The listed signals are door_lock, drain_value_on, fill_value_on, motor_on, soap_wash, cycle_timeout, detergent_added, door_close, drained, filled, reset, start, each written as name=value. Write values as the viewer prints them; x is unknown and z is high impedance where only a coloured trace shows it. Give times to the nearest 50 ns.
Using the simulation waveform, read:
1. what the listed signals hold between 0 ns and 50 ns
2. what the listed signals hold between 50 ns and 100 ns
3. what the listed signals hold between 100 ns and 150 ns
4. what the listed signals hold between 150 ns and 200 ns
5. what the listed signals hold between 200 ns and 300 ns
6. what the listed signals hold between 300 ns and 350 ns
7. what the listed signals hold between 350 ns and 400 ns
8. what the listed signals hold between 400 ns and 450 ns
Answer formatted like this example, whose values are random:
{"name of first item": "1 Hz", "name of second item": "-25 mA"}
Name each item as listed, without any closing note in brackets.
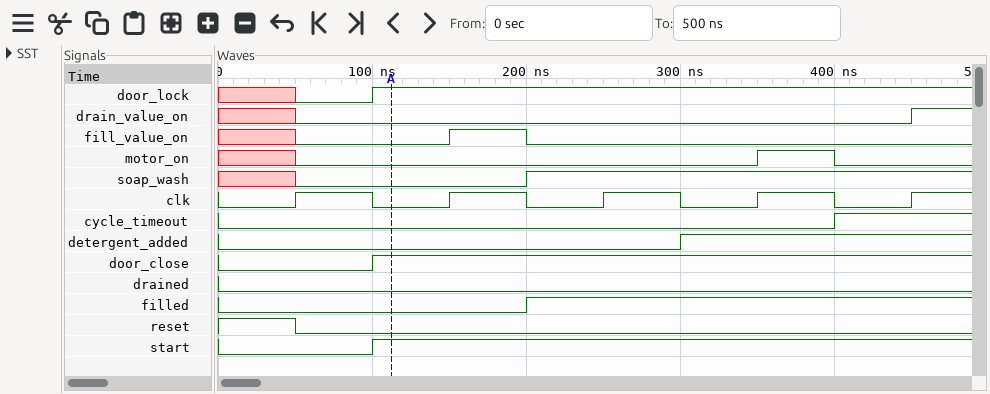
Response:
{"what the listed signals hold between 0 ns and 50 ns": "door_lock=x, drain_value_on=x, fill_value_on=x, motor_on=x, soap_wash=x, cycle_timeout=0, detergent_added=0, door_close=0, drained=0, filled=0, reset=1, start=0", "what the listed signals hold between 50 ns and 100 ns": "door_lock=0, drain_value_on=0, fill_value_on=0, motor_on=0, soap_wash=0, cycle_timeout=0, detergent_added=0, door_close=0, drained=0, filled=0, reset=0, start=0", "what the listed signals hold between 100 ns and 150 ns": "door_lock=1, drain_value_on=0, fill_value_on=0, motor_on=0, soap_wash=0, cycle_timeout=0, detergent_added=0, door_close=1, drained=0, filled=0, reset=0, start=1", "what the listed signals hold between 150 ns and 200 ns": "door_lock=1, drain_value_on=0, fill_value_on=1, motor_on=0, soap_wash=0, cycle_timeout=0, detergent_added=0, door_close=1, drained=0, filled=0, reset=0, start=1", "what the listed signals hold between 200 ns and 300 ns": "door_lock=1, drain_value_on=0, fill_value_on=0, motor_on=0, soap_wash=1, cycle_timeout=0, detergent_added=0, door_close=1, drained=0, filled=1, reset=0, start=1", "what the listed signals hold between 300 ns and 350 ns": "door_lock=1, drain_value_on=0, fill_value_on=0, motor_on=0, soap_wash=1, cycle_timeout=0, detergent_added=1, door_close=1, drained=0, filled=1, reset=0, start=1", "what the listed signals hold between 350 ns and 400 ns": "door_lock=1, drain_value_on=0, fill_value_on=0, motor_on=1, soap_wash=1, cycle_timeout=0, detergent_added=1, door_close=1, drained=0, filled=1, reset=0, start=1", "what the listed signals hold between 400 ns and 450 ns": "door_lock=1, drain_value_on=0, fill_value_on=0, motor_on=0, soap_wash=1, cycle_timeout=1, detergent_added=1, door_close=1, drained=0, filled=1, reset=0, start=1"}
